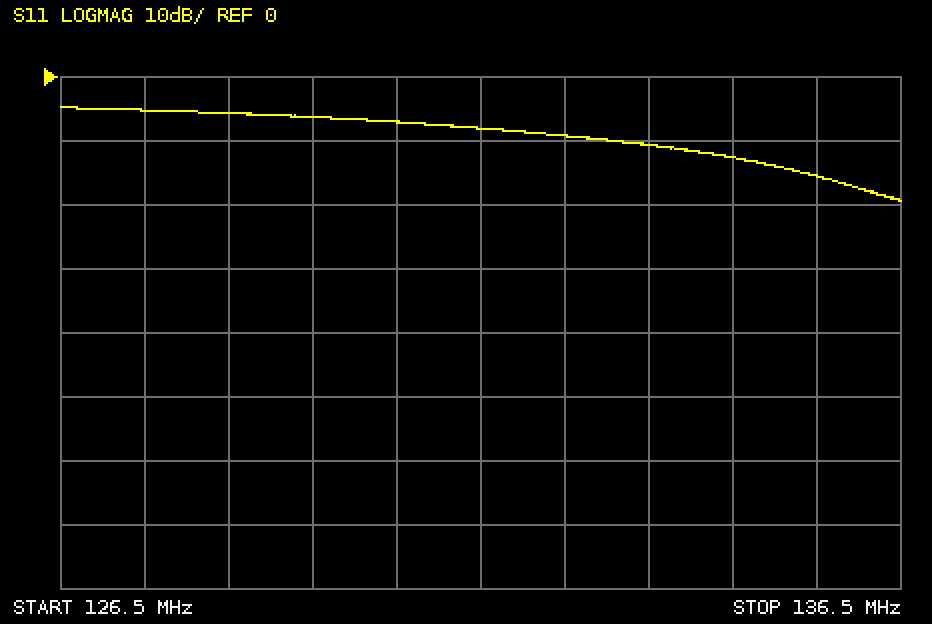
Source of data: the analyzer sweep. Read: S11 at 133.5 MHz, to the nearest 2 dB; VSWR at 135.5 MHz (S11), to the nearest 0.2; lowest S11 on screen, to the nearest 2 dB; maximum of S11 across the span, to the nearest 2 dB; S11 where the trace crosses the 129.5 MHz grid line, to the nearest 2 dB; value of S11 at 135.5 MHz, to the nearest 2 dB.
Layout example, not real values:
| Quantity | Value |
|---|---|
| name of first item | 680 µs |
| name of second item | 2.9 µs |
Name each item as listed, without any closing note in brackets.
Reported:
| Quantity | Value |
|---|---|
| S11 at 133.5 MHz, to the nearest 2 dB | -10 dB |
| VSWR at 135.5 MHz (S11), to the nearest 0.2 | 1.4 |
| lowest S11 on screen, to the nearest 2 dB | -20 dB |
| maximum of S11 across the span, to the nearest 2 dB | -4 dB |
| S11 where the trace crosses the 129.5 MHz grid line, to the nearest 2 dB | -6 dB |
| value of S11 at 135.5 MHz, to the nearest 2 dB | -16 dB |
